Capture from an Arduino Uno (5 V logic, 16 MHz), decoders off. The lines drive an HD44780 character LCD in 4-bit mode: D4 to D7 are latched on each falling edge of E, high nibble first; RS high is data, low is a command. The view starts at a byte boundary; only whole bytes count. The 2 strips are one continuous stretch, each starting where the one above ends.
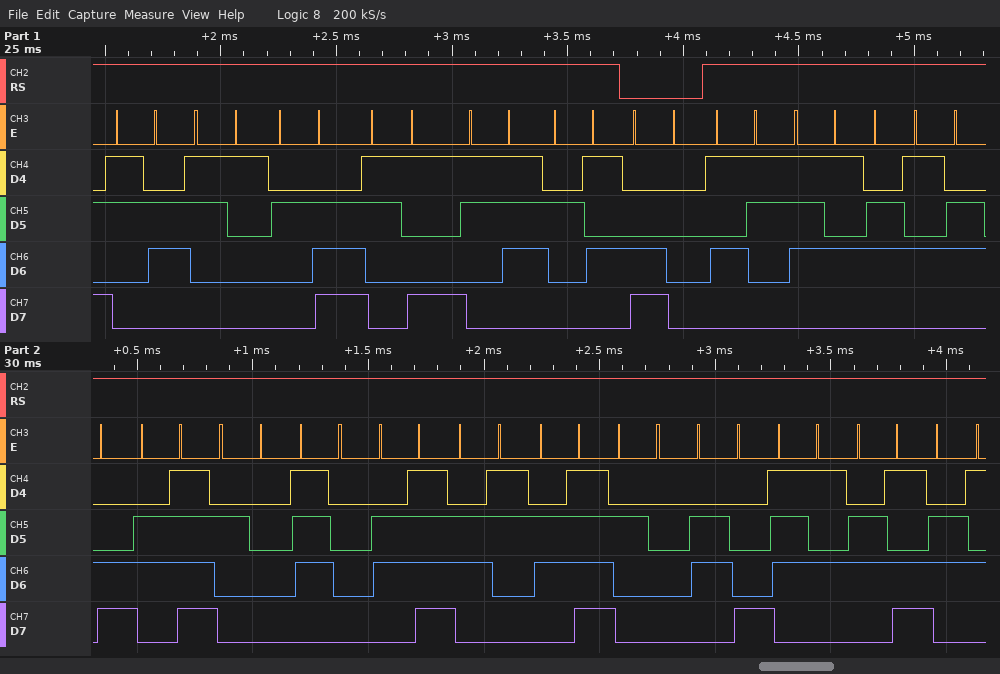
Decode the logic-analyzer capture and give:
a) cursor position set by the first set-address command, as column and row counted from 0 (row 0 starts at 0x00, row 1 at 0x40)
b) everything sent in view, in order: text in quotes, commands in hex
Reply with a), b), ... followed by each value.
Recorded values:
a) column 0, row 1
b) "61.97%" 0xC0 "Suelo poco hume"
